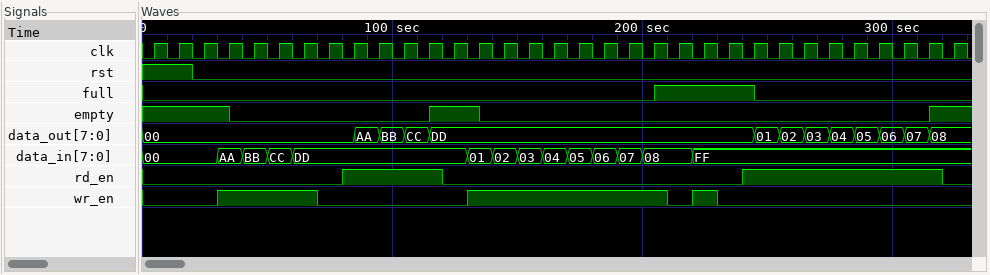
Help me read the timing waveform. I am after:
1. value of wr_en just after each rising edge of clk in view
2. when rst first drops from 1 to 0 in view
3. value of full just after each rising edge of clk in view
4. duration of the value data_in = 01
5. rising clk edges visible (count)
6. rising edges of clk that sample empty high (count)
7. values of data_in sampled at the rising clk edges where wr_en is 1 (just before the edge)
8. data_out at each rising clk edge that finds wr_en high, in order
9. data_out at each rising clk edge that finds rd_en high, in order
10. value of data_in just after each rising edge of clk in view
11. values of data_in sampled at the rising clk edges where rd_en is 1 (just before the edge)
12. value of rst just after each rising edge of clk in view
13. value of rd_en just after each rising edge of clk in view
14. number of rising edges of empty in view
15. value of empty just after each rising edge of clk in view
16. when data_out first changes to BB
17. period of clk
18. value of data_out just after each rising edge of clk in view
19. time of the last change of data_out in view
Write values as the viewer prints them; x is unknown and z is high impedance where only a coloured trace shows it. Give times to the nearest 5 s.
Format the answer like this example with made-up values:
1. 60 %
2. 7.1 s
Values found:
1. 0 0 0 1 1 1 1 0 0 0 0 0 0 1 1 1 1 1 1 1 1 0 1 0 0 0 0 0 0 0 0 0 0
2. 20 s
3. 0 0 0 0 0 0 0 0 0 0 0 0 0 0 0 0 0 0 0 0 1 1 1 1 0 0 0 0 0 0 0 0 0
4. 10 s
5. 33
6. 7
7. AA, BB, CC, DD, 01, 02, 03, 04, 05, 06, 07, 08, FF
8. 00, 00, 00, 00, DD, DD, DD, DD, DD, DD, DD, DD, DD
9. 00, AA, BB, CC, DD, 01, 02, 03, 04, 05, 06, 07
10. 00, 00, 00, AA, BB, CC, DD, DD, DD, DD, DD, DD, DD, 01, 02, 03, 04, 05, 06, 07, 08, 08, FF, FF, FF, FF, FF, FF, FF, FF, FF, FF, FF
11. DD, DD, DD, DD, FF, FF, FF, FF, FF, FF, FF, FF
12. 1 1 0 0 0 0 0 0 0 0 0 0 0 0 0 0 0 0 0 0 0 0 0 0 0 0 0 0 0 0 0 0 0
13. 0 0 0 0 0 0 0 0 1 1 1 1 0 0 0 0 0 0 0 0 0 0 0 0 1 1 1 1 1 1 1 1 0
14. 2
15. 1 1 1 0 0 0 0 0 0 0 0 1 1 0 0 0 0 0 0 0 0 0 0 0 0 0 0 0 0 0 0 1 1
16. 95 s
17. 10 s
18. 00, 00, 00, 00, 00, 00, 00, 00, AA, BB, CC, DD, DD, DD, DD, DD, DD, DD, DD, DD, DD, DD, DD, DD, 01, 02, 03, 04, 05, 06, 07, 08, 08
19. 315 s
